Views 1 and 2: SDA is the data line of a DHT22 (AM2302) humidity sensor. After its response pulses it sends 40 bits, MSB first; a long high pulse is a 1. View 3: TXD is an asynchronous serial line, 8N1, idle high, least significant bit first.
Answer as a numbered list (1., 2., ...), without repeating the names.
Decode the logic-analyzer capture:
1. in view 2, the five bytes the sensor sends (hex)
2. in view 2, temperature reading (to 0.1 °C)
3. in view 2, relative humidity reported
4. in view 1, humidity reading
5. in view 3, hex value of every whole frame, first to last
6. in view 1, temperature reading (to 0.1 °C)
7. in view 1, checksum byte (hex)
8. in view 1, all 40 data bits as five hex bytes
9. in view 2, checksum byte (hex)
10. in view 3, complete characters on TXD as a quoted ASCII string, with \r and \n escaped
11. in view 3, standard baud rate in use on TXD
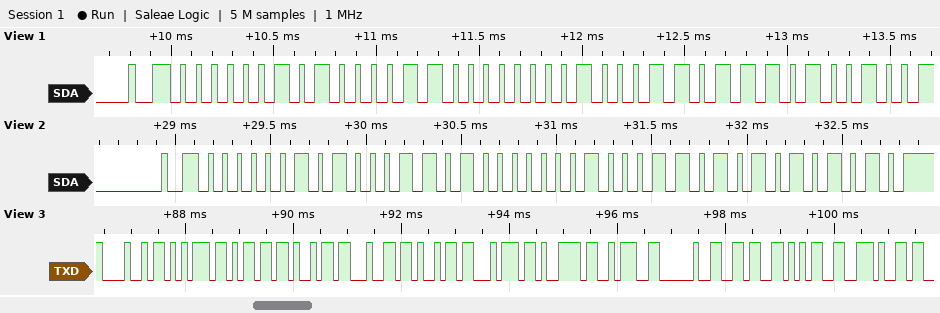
1. 02 8D 01 1A AA
2. 28.2 °C
3. 65.3 %
4. 64.6 %
5. 48 75 6D 69 64 69 74 79 3A 20 36 35 2E
6. 28.3 °C
7. 0xA4
8. 02 86 01 1B A4
9. 0xAA
10. "Humidity: 65."
11. 9600 baud
